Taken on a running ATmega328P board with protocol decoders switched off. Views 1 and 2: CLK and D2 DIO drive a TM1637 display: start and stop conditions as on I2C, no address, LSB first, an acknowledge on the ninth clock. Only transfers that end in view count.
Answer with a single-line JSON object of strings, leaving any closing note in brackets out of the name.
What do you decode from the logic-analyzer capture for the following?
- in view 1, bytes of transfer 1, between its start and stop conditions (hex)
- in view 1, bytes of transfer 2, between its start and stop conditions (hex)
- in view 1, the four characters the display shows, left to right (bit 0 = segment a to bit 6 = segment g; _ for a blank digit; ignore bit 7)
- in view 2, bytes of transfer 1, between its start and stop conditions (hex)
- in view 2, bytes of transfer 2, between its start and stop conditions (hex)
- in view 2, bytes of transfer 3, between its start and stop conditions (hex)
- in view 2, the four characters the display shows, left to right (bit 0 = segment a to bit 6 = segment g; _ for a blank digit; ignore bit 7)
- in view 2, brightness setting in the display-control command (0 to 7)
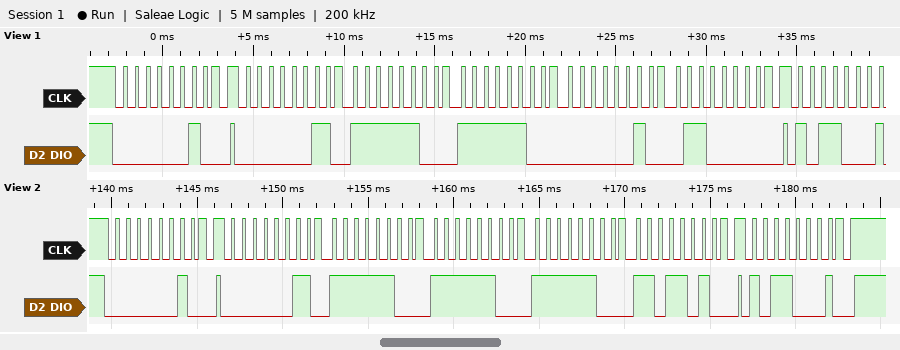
{"in view 1, bytes of transfer 1, between its start and stop conditions": "40", "in view 1, bytes of transfer 2, between its start and stop conditions": "C0 3F 3F 40 06", "in view 1, the four characters the display shows, left to right": "00-1", "in view 2, bytes of transfer 1, between its start and stop conditions": "40", "in view 2, bytes of transfer 2, between its start and stop conditions": "C0 3F 3F 3F 5B", "in view 2, bytes of transfer 3, between its start and stop conditions": "8D", "in view 2, the four characters the display shows, left to right": "0002", "in view 2, brightness setting in the display-control command": "5"}
